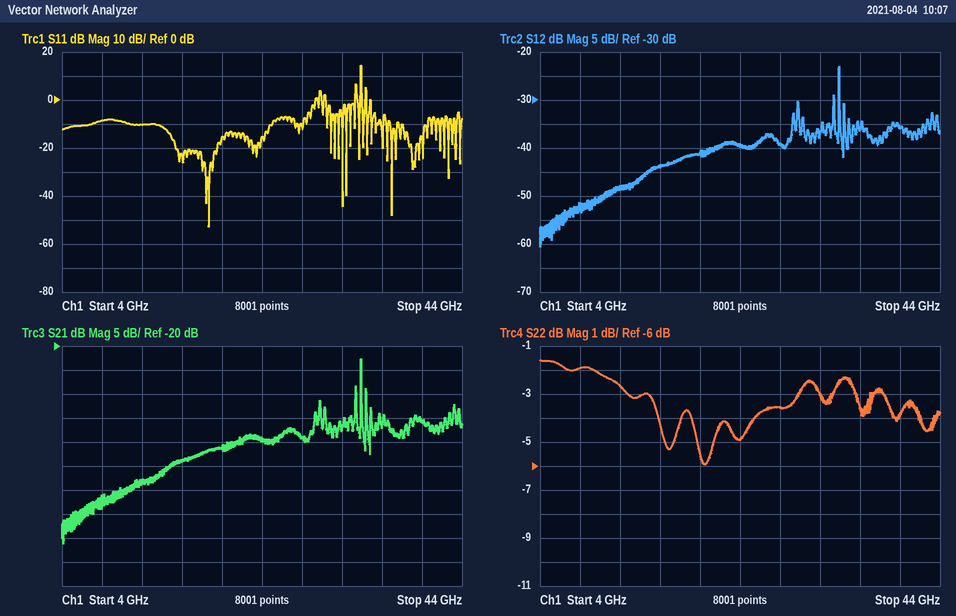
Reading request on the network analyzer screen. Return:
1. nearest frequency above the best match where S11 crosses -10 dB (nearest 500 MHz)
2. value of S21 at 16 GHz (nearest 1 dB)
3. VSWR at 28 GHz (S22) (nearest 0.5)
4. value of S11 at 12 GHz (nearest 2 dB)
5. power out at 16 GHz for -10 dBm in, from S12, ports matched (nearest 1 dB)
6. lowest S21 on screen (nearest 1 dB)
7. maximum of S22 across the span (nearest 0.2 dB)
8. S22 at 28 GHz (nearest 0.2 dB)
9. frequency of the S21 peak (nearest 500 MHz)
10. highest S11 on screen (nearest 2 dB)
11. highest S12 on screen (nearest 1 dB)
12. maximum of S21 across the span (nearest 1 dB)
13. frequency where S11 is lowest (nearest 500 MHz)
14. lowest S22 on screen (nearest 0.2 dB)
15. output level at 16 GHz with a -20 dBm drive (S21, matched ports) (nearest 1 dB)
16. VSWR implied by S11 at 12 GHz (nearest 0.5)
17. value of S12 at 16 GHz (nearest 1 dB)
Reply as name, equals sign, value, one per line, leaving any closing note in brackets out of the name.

nearest frequency above the best match where S11 crosses -10 dB = 25.0 GHz
value of S21 at 16 GHz = -44 dB
VSWR at 28 GHz (S22) = 5.0
value of S11 at 12 GHz = -10 dB
power out at 16 GHz for -10 dBm in, from S12, ports matched = -54 dBm
lowest S21 on screen = -61 dB
maximum of S22 across the span = -1.6 dB
S22 at 28 GHz = -3.6 dB
frequency of the S21 peak = 34.0 GHz
highest S11 on screen = 14 dB
highest S12 on screen = -23 dB
maximum of S21 across the span = -23 dB
frequency where S11 is lowest = 18.5 GHz
lowest S22 on screen = -6.0 dB
output level at 16 GHz with a -20 dBm drive (S21, matched ports) = -64 dBm
VSWR implied by S11 at 12 GHz = 2.0
value of S12 at 16 GHz = -44 dB
